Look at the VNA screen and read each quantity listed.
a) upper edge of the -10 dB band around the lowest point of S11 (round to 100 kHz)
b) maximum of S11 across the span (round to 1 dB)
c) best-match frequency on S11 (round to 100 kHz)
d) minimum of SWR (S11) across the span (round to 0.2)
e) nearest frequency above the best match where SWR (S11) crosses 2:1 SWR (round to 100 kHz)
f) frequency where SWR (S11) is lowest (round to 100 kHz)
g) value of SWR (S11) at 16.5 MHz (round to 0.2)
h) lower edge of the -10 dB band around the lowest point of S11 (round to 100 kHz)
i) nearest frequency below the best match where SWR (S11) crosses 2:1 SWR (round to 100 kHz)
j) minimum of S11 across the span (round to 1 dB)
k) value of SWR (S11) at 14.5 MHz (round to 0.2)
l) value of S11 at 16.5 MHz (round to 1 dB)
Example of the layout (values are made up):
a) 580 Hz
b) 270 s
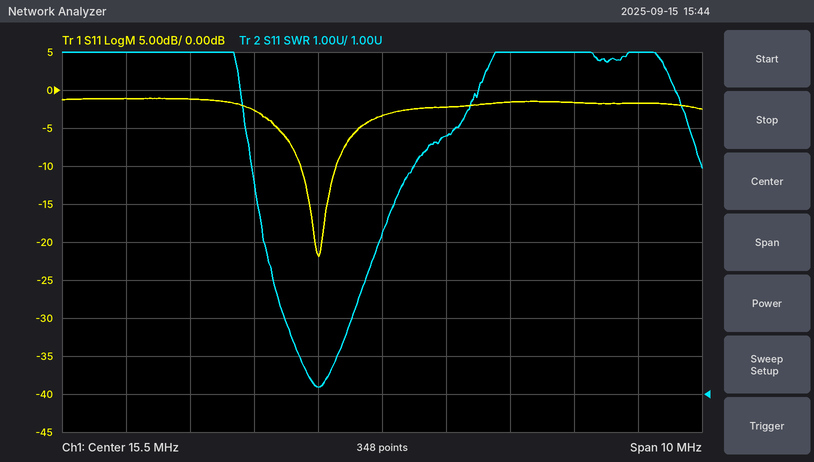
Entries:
a) 14.8 MHz
b) -1 dB
c) 14.5 MHz
d) 1.2
e) 14.8 MHz
f) 14.5 MHz
g) 7.8
h) 14.2 MHz
i) 14.2 MHz
j) -22 dB
k) 1.2
l) -2 dB
